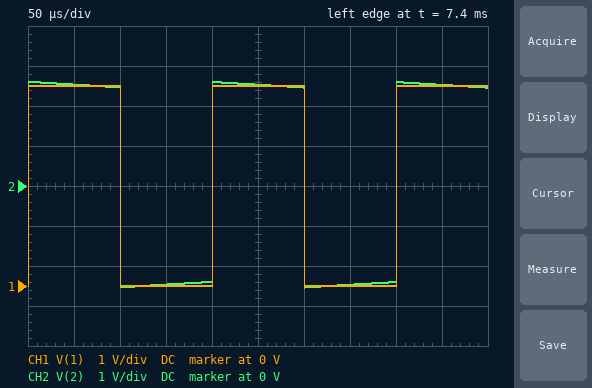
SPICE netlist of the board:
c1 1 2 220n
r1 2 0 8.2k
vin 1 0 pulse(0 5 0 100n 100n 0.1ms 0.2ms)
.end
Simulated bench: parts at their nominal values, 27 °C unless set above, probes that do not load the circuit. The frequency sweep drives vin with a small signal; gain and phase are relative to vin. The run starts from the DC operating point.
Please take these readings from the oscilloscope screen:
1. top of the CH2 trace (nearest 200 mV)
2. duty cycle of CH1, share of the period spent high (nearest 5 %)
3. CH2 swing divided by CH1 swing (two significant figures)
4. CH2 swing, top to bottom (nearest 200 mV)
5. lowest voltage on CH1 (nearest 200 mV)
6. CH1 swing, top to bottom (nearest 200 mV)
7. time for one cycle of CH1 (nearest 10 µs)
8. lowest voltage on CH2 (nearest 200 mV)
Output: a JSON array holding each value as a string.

["2.6 V", "50 %", "1.0", "5.2 V", "0 V", "5.0 V", "200 µs", "-2.6 V"]
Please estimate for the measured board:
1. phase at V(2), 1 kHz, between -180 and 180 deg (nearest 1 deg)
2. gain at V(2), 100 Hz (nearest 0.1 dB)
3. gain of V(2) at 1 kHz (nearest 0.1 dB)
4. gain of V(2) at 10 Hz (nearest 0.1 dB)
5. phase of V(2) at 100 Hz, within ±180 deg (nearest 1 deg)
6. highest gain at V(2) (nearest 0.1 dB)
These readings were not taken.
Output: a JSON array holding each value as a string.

["5 deg", "-2.5 dB", "0 dB", "-19.0 dB", "41 deg", "0 dB"]
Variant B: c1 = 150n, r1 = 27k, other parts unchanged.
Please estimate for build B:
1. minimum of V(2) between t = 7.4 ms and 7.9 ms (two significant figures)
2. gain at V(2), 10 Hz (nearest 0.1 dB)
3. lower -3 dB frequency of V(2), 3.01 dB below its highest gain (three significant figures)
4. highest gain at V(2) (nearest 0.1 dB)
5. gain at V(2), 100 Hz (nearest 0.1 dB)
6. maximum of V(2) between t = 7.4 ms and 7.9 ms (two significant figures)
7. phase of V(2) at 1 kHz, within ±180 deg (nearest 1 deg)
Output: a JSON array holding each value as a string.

["-2.2 V", "-12.2 dB", "39.3 Hz", "0 dB", "-0.6 dB", "2.9 V", "2 deg"]
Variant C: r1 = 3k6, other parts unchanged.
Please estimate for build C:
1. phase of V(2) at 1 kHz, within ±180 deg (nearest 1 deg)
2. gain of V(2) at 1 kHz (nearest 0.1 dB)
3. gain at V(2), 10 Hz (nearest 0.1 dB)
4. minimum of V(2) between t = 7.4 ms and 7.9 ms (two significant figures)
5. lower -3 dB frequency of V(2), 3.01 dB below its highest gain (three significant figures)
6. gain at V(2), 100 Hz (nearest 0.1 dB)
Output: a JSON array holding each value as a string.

["11 deg", "-0.2 dB", "-26.1 dB", "-2.7 V", "201 Hz", "-7.0 dB"]
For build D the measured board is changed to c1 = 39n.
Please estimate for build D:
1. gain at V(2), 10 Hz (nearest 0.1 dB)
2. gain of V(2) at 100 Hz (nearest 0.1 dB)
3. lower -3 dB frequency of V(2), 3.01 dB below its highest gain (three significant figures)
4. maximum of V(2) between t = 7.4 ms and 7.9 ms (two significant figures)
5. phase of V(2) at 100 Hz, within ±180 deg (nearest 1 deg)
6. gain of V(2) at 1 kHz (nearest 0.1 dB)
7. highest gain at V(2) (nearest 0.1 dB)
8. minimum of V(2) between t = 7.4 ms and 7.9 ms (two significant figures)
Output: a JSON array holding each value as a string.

["-33.9 dB", "-14.1 dB", "498 Hz", "2.9 V", "79 deg", "-1.0 dB", "0 dB", "-2.9 V"]
